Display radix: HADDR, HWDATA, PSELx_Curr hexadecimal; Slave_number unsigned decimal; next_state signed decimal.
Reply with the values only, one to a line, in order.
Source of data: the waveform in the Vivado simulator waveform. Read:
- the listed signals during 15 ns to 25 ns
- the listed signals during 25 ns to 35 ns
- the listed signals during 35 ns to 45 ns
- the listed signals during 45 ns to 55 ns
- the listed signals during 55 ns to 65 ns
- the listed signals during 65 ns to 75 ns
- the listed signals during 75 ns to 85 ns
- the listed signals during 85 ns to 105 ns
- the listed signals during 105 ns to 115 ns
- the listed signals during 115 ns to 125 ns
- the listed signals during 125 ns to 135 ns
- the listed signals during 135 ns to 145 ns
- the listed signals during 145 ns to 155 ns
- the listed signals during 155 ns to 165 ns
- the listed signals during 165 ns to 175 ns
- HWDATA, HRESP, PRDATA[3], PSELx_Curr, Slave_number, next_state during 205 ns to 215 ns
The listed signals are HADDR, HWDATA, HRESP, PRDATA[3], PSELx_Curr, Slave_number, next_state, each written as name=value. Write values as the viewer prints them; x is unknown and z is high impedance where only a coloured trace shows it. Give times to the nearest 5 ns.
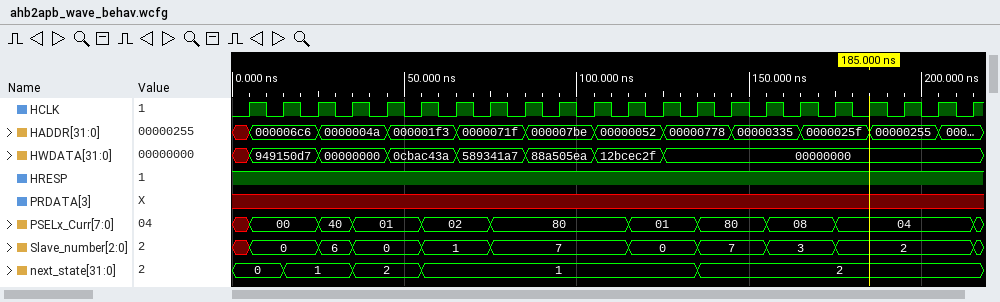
HADDR=000006c6, HWDATA=949150d7, HRESP=1, PRDATA[3]=x, PSELx_Curr=00, Slave_number=0, next_state=1
HADDR=0000004a, HWDATA=00000000, HRESP=1, PRDATA[3]=x, PSELx_Curr=40, Slave_number=6, next_state=1
HADDR=0000004a, HWDATA=00000000, HRESP=1, PRDATA[3]=x, PSELx_Curr=01, Slave_number=0, next_state=2
HADDR=000001f3, HWDATA=0cbac43a, HRESP=1, PRDATA[3]=x, PSELx_Curr=01, Slave_number=0, next_state=2
HADDR=000001f3, HWDATA=0cbac43a, HRESP=1, PRDATA[3]=x, PSELx_Curr=02, Slave_number=1, next_state=1
HADDR=0000071f, HWDATA=589341a7, HRESP=1, PRDATA[3]=x, PSELx_Curr=02, Slave_number=1, next_state=1
HADDR=0000071f, HWDATA=589341a7, HRESP=1, PRDATA[3]=x, PSELx_Curr=80, Slave_number=7, next_state=1
HADDR=000007be, HWDATA=88a505ea, HRESP=1, PRDATA[3]=x, PSELx_Curr=80, Slave_number=7, next_state=1
HADDR=00000052, HWDATA=12bcec2f, HRESP=1, PRDATA[3]=x, PSELx_Curr=80, Slave_number=7, next_state=1
HADDR=00000052, HWDATA=12bcec2f, HRESP=1, PRDATA[3]=x, PSELx_Curr=01, Slave_number=0, next_state=1
HADDR=00000778, HWDATA=00000000, HRESP=1, PRDATA[3]=x, PSELx_Curr=01, Slave_number=0, next_state=1
HADDR=00000778, HWDATA=00000000, HRESP=1, PRDATA[3]=x, PSELx_Curr=80, Slave_number=7, next_state=2
HADDR=00000335, HWDATA=00000000, HRESP=1, PRDATA[3]=x, PSELx_Curr=80, Slave_number=7, next_state=2
HADDR=00000335, HWDATA=00000000, HRESP=1, PRDATA[3]=x, PSELx_Curr=08, Slave_number=3, next_state=2
HADDR=0000025f, HWDATA=00000000, HRESP=1, PRDATA[3]=x, PSELx_Curr=08, Slave_number=3, next_state=2
HWDATA=00000000, HRESP=1, PRDATA[3]=x, PSELx_Curr=04, Slave_number=2, next_state=2
